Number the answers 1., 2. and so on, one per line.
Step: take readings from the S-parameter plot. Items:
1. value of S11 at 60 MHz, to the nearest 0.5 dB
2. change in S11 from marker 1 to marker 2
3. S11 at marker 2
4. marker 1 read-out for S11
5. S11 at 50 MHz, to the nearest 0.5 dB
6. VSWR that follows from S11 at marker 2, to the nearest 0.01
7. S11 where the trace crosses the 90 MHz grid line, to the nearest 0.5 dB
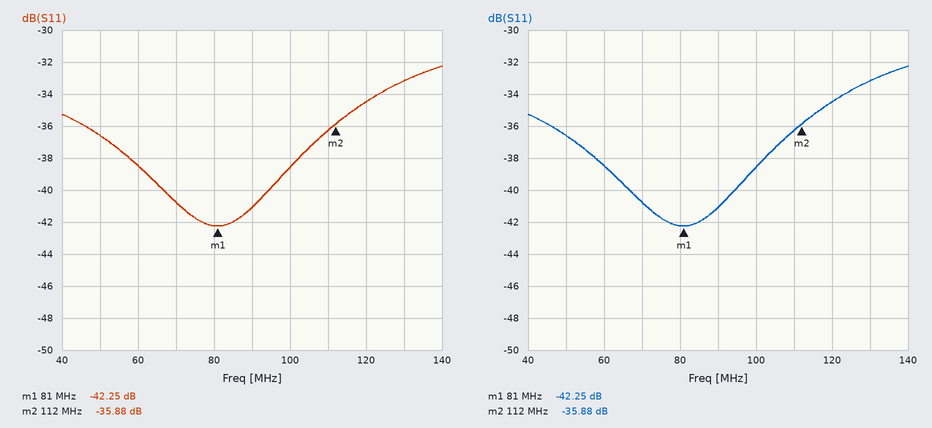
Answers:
1. -38.5 dB
2. 6.37 dB
3. -35.88 dB
4. -42.25 dB
5. -36.5 dB
6. 1.03
7. -41.0 dB
